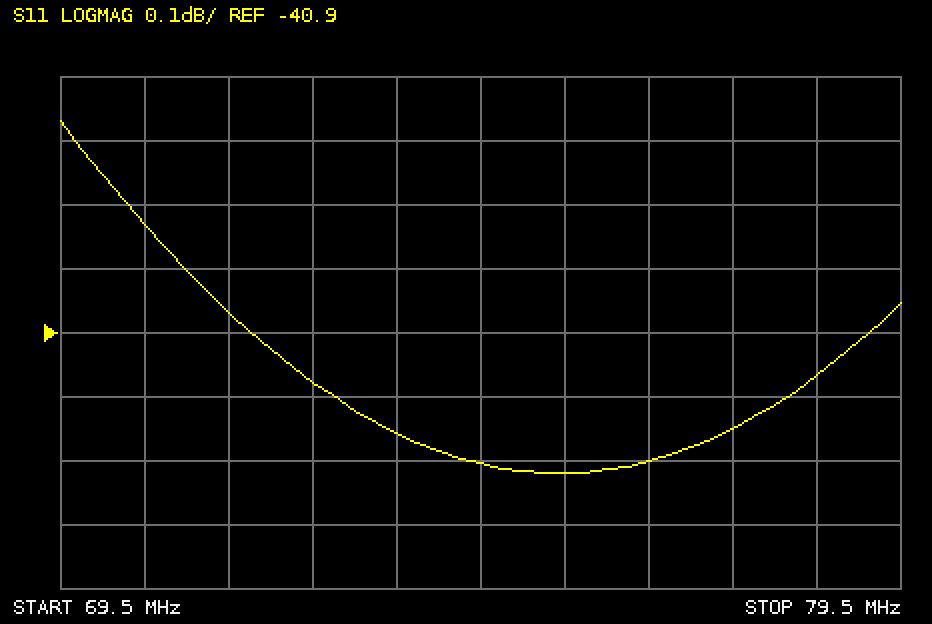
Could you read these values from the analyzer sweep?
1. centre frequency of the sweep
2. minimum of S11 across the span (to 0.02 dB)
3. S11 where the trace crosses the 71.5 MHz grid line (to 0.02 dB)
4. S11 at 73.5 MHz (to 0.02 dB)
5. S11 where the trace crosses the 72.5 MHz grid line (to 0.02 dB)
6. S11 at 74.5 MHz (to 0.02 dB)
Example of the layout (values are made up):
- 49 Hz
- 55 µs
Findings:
- 74.5 MHz
- -41.12 dB
- -40.86 dB
- -41.06 dB
- -40.98 dB
- -41.10 dB
